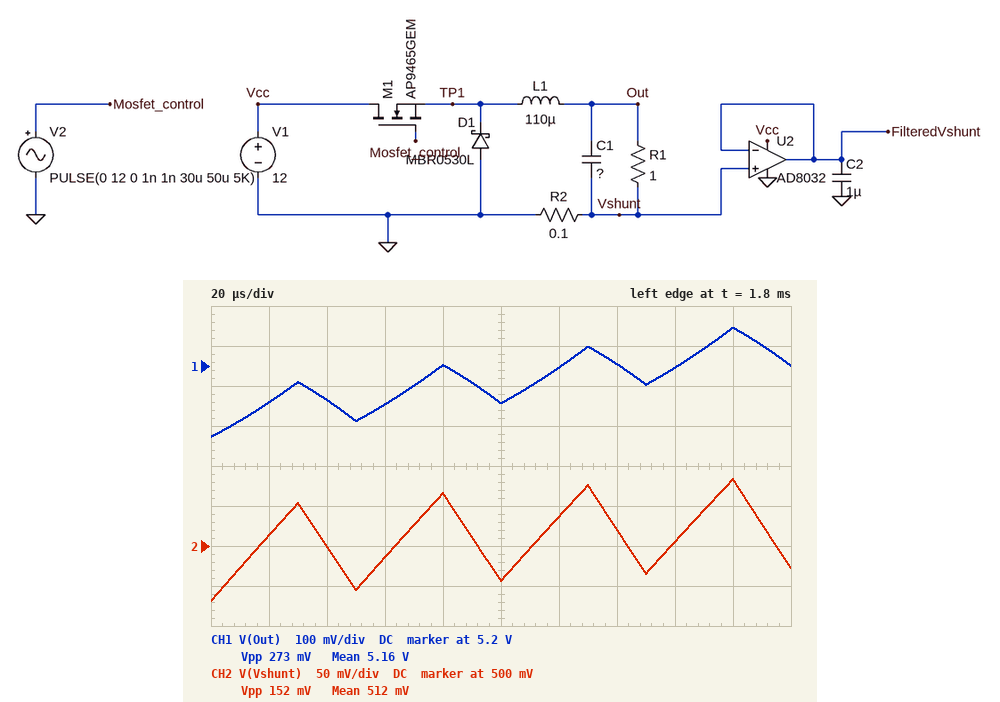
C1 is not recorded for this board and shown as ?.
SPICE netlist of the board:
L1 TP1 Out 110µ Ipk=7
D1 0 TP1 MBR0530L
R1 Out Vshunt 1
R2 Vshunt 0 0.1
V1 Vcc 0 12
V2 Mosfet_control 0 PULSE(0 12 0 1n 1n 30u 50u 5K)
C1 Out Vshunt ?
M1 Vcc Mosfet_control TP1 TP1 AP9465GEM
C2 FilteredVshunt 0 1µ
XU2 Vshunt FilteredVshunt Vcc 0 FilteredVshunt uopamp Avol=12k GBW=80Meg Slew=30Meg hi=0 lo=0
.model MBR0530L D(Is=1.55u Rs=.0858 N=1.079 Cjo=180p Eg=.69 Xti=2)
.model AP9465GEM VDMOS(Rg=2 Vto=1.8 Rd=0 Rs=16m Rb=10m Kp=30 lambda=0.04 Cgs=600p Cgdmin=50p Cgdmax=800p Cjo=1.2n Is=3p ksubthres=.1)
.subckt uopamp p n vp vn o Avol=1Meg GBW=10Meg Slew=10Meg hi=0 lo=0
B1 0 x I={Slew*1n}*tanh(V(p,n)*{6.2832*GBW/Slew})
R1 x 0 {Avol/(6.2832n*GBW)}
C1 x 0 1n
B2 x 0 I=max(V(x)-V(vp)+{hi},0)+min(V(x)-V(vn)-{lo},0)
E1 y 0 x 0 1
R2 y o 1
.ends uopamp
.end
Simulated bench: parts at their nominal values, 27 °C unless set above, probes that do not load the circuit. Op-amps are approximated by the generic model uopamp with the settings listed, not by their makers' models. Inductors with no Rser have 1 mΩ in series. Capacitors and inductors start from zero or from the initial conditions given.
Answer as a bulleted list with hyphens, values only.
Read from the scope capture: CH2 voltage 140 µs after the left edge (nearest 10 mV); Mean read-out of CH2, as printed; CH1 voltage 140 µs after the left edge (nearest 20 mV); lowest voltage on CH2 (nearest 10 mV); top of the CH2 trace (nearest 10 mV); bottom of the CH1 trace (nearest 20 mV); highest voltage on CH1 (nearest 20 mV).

- 520 mV
- 512 mV
- 5.20 V
- 430 mV
- 580 mV
- 5.02 V
- 5.30 V
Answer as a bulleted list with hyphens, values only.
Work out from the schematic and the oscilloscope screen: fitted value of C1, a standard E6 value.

- 680 µF
